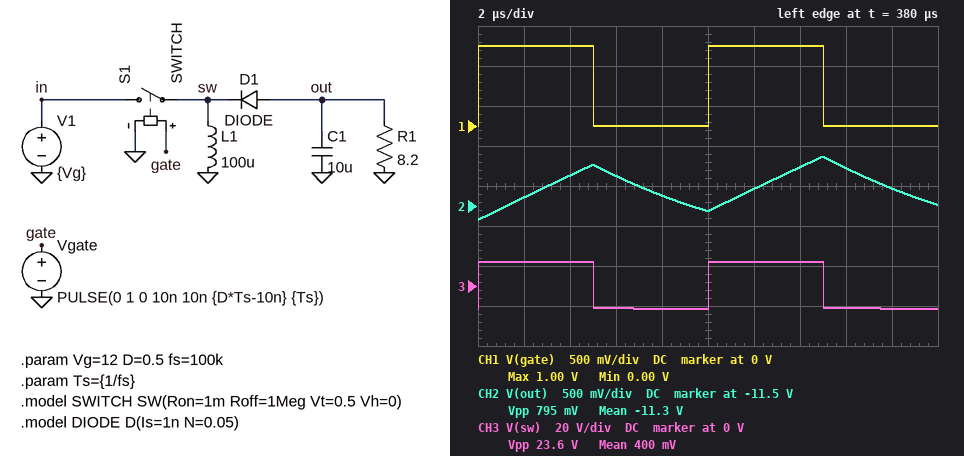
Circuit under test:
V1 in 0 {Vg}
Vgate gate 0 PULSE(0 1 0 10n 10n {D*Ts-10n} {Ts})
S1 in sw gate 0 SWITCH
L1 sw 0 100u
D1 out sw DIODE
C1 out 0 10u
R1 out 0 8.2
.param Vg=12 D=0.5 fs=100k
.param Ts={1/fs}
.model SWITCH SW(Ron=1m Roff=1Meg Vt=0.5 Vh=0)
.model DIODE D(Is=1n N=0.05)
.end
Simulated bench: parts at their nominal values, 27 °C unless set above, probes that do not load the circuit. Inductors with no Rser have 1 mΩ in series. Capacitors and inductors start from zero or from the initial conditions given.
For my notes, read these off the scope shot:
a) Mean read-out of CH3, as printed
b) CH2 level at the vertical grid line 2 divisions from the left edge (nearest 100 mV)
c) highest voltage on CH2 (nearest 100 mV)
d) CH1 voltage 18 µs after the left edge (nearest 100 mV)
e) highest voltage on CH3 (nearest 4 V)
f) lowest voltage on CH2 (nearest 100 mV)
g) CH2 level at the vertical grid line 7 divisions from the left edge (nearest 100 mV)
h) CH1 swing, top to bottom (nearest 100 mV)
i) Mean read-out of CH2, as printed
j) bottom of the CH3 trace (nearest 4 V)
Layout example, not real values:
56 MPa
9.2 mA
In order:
400 mV
-11.1 V
-10.9 V
0 V
12 V
-11.7 V
-11.0 V
1.0 V
-11.3 V
-12 V
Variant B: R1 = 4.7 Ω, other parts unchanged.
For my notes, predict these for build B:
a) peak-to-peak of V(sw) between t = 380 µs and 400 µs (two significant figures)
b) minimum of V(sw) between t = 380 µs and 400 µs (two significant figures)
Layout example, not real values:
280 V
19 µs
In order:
25 V
-13 V
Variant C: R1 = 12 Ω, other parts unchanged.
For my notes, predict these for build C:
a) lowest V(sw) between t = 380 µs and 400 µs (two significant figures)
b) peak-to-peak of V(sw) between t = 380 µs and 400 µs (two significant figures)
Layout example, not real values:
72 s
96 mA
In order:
-10 V
22 V
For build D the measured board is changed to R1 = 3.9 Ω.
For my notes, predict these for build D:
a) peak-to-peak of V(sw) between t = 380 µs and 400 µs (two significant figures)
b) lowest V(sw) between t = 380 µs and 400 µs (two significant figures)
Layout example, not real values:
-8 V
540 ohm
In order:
25 V
-13 V
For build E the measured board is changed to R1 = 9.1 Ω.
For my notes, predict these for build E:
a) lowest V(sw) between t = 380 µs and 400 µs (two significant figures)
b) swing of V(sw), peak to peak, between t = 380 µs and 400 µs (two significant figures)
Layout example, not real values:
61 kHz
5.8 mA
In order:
-11 V
23 V
